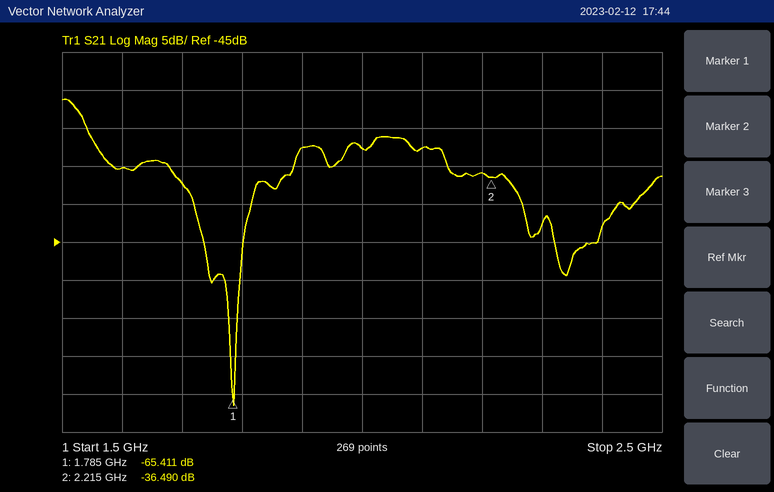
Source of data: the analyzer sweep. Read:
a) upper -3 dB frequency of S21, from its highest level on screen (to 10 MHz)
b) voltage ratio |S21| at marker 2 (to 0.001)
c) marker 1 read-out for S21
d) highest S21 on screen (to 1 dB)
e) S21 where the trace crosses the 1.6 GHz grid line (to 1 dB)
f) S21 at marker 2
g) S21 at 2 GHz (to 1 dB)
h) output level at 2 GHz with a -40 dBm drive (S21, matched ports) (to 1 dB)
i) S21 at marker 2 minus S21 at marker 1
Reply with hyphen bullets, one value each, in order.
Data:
- 1.54 GHz
- 0.015
- -65.411 dB
- -26 dB
- -35 dB
- -36.490 dB
- -33 dB
- -73 dBm
- 28.921 dB
